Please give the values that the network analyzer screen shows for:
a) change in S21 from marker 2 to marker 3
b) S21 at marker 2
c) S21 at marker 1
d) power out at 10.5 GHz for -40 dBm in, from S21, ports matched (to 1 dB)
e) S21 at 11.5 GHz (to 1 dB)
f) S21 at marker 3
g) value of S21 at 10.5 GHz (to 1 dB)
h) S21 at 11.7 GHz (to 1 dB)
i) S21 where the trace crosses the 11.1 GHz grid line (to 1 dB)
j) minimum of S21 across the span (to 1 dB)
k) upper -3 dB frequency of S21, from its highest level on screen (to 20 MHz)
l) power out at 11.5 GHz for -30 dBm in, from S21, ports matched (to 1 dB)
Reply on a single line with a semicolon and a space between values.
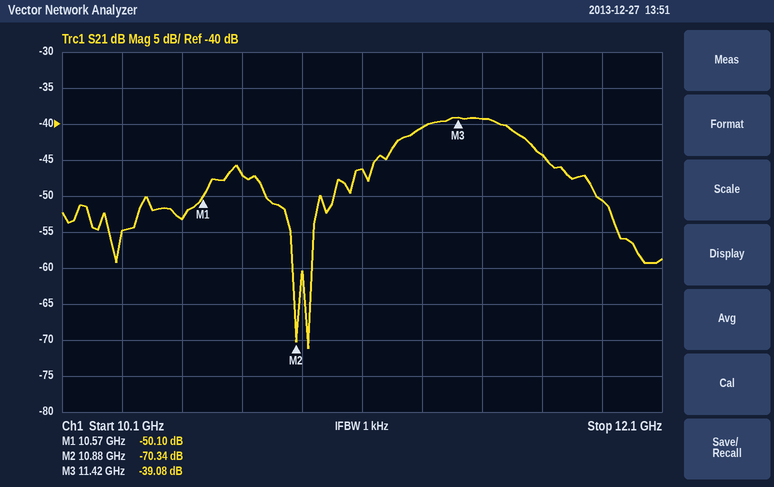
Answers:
31.26 dB; -70.34 dB; -50.10 dB; -93 dBm; -39 dB; -39.08 dB; -53 dB; -44 dB; -46 dB; -71 dB; 11.64 GHz; -69 dBm
